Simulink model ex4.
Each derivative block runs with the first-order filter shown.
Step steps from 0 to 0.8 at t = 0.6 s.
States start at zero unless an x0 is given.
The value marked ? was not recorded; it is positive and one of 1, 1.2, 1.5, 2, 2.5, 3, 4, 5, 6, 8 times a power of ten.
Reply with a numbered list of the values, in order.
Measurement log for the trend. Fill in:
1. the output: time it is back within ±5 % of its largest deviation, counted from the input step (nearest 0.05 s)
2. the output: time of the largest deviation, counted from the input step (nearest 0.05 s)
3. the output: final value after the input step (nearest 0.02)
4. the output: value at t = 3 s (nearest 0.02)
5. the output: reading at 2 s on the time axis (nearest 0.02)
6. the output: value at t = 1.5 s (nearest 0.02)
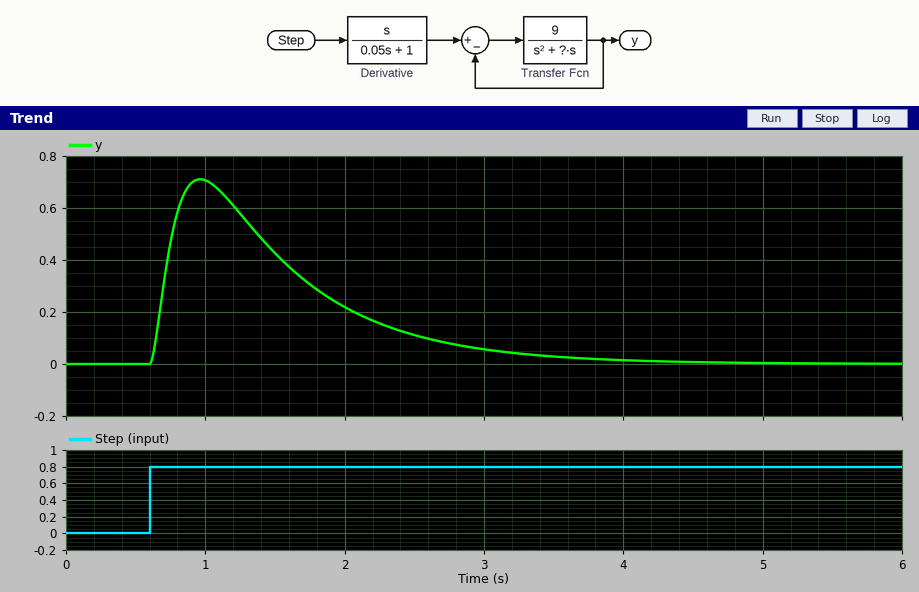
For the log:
1. 2.75 s
2. 0.35 s
3. 0.00
4. 0.06
5. 0.22
6. 0.42
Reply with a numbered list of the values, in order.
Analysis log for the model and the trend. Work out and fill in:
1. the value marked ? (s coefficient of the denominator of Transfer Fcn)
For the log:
1. 8
